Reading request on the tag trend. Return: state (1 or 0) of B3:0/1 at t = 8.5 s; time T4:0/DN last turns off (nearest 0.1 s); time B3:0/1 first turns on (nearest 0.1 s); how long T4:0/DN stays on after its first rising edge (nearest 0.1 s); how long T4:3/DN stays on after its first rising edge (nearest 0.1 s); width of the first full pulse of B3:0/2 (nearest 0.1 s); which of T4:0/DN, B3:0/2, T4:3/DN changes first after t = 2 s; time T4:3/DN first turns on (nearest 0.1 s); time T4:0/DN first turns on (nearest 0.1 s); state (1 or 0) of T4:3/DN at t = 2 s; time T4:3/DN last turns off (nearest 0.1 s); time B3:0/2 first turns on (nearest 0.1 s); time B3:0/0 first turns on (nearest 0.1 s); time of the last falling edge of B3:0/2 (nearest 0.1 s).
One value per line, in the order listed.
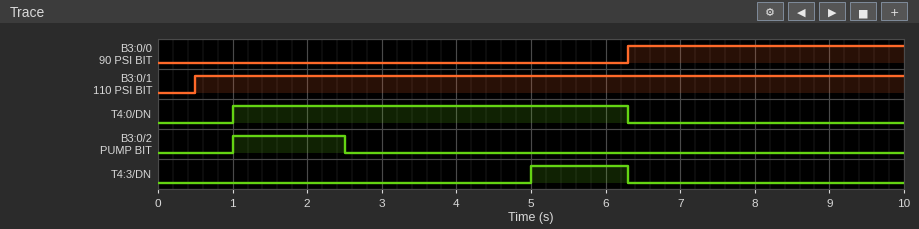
1
6.3 s
0.5 s
5.3 s
1.3 s
1.5 s
B3:0/2
5.0 s
1.0 s
0
6.3 s
1.0 s
6.3 s
2.5 s
